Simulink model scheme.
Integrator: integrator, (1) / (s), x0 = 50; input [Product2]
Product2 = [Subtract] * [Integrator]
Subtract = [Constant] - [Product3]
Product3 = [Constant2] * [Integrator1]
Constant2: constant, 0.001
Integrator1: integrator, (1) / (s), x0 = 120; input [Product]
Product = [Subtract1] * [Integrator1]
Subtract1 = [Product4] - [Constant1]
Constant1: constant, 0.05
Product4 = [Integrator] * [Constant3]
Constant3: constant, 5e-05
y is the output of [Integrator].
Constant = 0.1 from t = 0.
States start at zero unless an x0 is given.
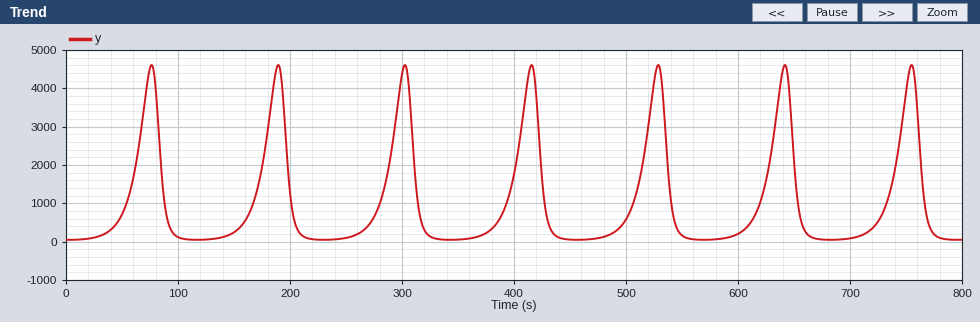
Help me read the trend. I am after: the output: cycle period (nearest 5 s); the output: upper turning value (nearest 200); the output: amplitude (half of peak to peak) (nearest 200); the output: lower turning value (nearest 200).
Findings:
115 s
4600
2200
0
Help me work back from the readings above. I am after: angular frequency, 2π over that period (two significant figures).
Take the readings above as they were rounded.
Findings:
0.055 rad/s
